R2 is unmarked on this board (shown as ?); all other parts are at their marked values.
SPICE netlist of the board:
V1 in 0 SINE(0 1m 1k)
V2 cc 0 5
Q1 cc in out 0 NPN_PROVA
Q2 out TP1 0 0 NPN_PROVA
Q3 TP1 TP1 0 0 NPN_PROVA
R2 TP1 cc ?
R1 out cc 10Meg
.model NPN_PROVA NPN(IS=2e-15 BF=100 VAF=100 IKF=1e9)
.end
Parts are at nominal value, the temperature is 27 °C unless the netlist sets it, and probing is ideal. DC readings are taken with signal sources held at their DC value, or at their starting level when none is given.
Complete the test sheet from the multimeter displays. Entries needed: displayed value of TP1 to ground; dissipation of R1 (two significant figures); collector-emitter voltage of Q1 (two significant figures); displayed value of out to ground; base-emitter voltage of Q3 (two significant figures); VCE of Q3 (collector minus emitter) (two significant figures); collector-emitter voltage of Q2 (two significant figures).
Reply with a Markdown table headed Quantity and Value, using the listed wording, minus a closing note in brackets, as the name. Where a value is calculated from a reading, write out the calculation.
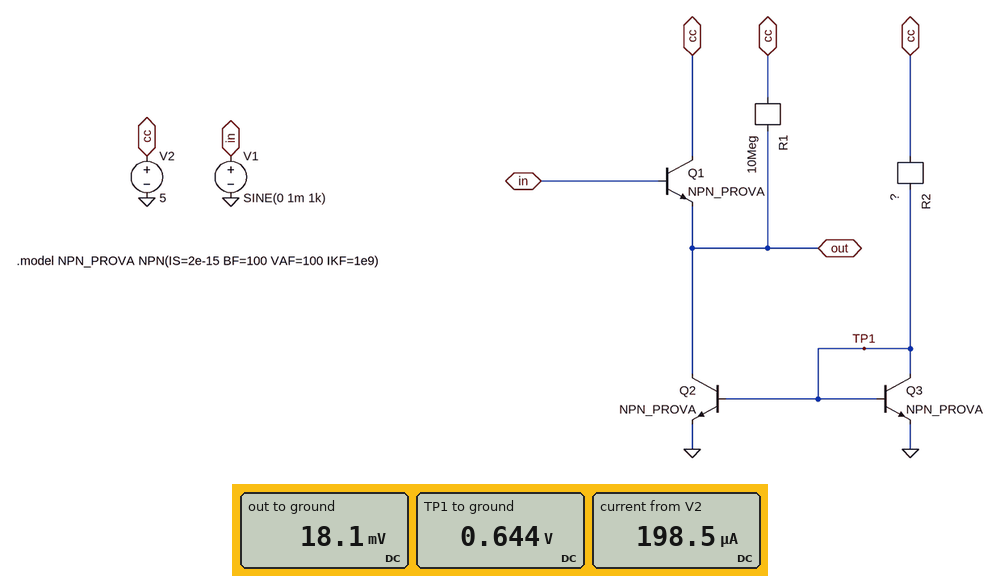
| Quantity | Value |
|---|---|
| displayed value of TP1 to ground | 0.644 V |
| dissipation of R1 | (5 V - 18.1 mV)^2 / 10 MΩ = 2.5 µW |
| collector-emitter voltage of Q1 | 5 V - 18.1 mV = 5.0 V |
| displayed value of out to ground | 18.1 mV |
| base-emitter voltage of Q3 | 644 mV = 640 mV |
| VCE of Q3 (collector minus emitter) | 644 mV = 640 mV |
| collector-emitter voltage of Q2 | 18.1 mV = 18 mV |
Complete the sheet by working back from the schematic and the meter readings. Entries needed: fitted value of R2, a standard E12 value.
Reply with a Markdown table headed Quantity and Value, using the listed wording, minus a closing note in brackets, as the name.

| Quantity | Value |
|---|---|
| fitted value of R2, a standard E12 value | 22 kΩ |
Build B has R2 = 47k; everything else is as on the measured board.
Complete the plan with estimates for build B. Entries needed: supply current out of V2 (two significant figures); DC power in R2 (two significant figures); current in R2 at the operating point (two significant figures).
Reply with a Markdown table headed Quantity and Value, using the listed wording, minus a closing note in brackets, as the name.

| Quantity | Value |
|---|---|
| supply current out of V2 | 94 µA |
| DC power in R2 | 410 µW |
| current in R2 at the operating point | 93 µA |
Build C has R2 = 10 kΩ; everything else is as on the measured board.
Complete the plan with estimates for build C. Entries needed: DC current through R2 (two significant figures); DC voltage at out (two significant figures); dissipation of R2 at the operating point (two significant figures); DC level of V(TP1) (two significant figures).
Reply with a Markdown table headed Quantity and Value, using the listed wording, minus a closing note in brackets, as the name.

| Quantity | Value |
|---|---|
| DC current through R2 | 430 µA |
| DC voltage at out | 18 mV |
| dissipation of R2 at the operating point | 1.9 mW |
| DC level of V(TP1) | 660 mV |
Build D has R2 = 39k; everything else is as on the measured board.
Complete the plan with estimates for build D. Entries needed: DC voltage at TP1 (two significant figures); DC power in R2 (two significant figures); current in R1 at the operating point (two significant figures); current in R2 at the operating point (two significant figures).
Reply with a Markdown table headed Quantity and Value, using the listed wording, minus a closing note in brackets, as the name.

| Quantity | Value |
|---|---|
| DC voltage at TP1 | 630 mV |
| DC power in R2 | 490 µW |
| current in R1 at the operating point | 500 nA |
| current in R2 at the operating point | 110 µA |
